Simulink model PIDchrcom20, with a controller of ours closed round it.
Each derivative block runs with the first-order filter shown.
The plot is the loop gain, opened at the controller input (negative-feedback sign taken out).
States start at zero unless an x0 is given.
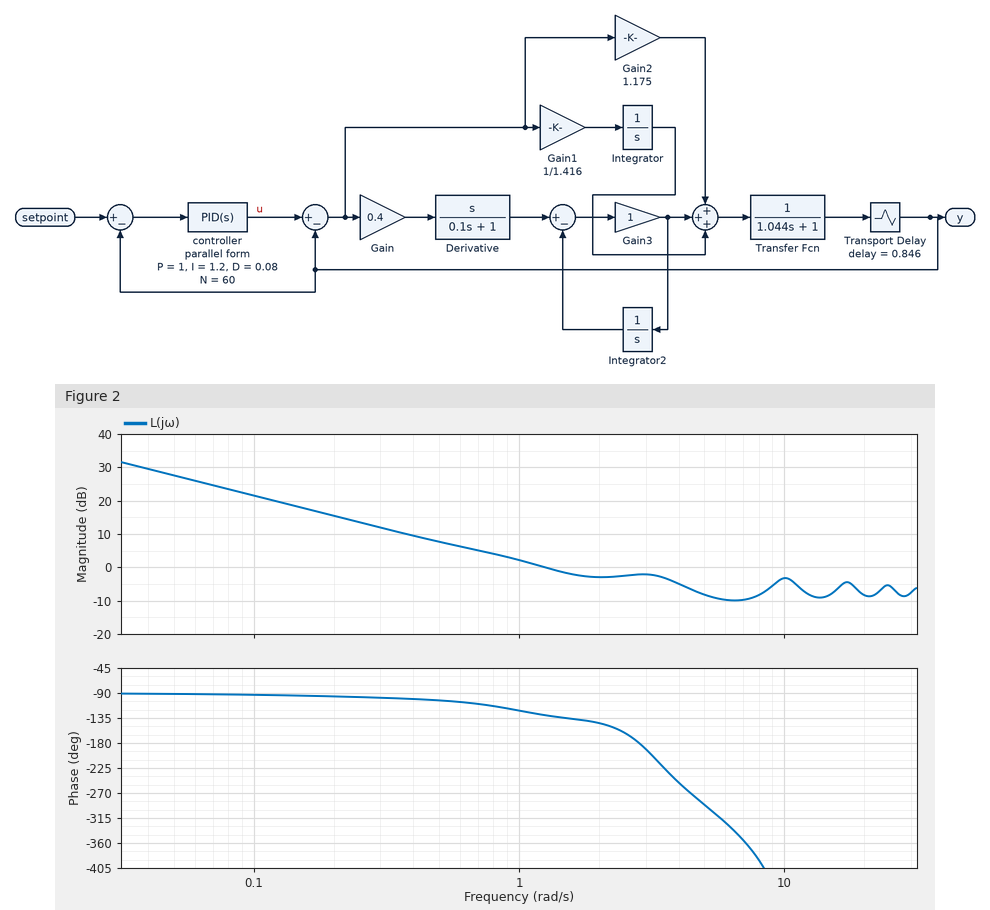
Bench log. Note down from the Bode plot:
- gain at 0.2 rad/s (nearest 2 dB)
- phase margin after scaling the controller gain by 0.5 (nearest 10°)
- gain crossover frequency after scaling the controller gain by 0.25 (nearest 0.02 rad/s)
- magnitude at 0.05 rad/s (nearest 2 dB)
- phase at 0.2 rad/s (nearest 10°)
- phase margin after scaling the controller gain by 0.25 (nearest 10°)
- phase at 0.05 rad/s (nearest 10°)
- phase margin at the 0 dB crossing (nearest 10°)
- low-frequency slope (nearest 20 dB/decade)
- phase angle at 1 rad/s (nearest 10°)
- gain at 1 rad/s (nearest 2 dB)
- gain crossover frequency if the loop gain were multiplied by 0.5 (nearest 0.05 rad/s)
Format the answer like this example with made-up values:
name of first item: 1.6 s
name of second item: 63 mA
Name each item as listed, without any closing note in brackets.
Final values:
gain at 0.2 rad/s: 16 dB
phase margin after scaling the controller gain by 0.5: 70°
gain crossover frequency after scaling the controller gain by 0.25: 0.30 rad/s
magnitude at 0.05 rad/s: 28 dB
phase at 0.2 rad/s: -100°
phase margin after scaling the controller gain by 0.25: 80°
phase at 0.05 rad/s: -90°
phase margin at the 0 dB crossing: 50°
low-frequency slope: -20 dB/decade
phase angle at 1 rad/s: -120°
gain at 1 rad/s: 2 dB
gain crossover frequency if the loop gain were multiplied by 0.5: 0.60 rad/s
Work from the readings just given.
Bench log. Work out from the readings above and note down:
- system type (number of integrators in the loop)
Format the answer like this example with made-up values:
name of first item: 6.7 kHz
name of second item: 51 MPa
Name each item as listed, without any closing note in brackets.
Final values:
system type: 1
